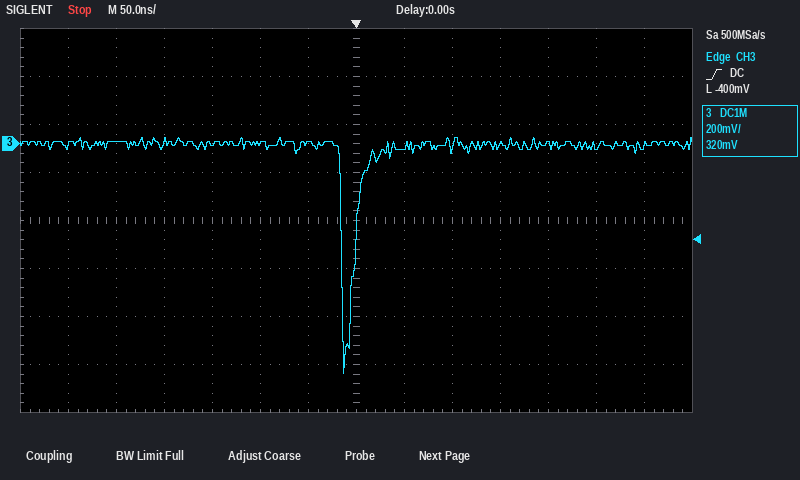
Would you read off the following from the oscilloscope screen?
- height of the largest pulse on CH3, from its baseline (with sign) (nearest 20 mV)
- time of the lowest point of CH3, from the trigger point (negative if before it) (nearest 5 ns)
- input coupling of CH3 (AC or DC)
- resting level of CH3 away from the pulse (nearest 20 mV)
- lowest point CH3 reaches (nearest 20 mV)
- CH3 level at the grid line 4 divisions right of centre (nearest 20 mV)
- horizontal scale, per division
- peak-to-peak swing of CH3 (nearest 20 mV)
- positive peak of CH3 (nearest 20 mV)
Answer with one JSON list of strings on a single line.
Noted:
["-960 mV", "-15 ns", "DC", "0 mV", "-960 mV", "0 mV", "50 ns", "980 mV", "20 mV"]
